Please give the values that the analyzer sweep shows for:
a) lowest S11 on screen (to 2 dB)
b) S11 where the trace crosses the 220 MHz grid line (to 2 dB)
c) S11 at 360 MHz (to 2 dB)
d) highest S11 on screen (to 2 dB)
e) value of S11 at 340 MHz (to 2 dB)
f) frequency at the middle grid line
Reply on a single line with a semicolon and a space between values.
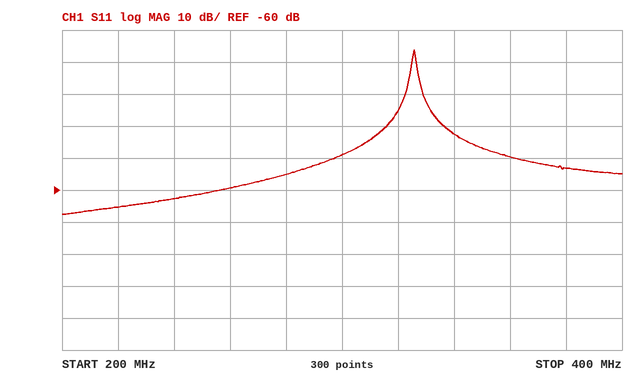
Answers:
-68 dB; -66 dB; -50 dB; -16 dB; -42 dB; 300 MHz
